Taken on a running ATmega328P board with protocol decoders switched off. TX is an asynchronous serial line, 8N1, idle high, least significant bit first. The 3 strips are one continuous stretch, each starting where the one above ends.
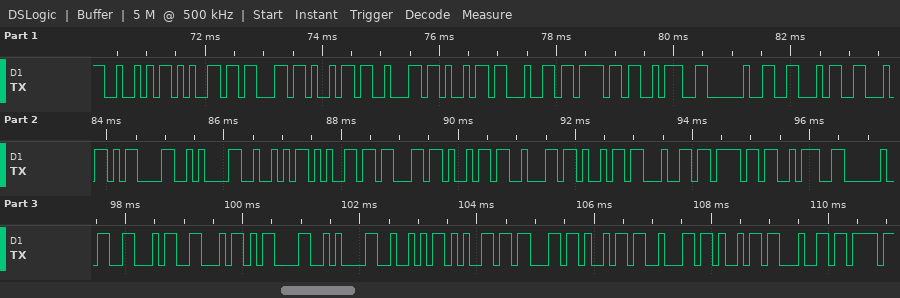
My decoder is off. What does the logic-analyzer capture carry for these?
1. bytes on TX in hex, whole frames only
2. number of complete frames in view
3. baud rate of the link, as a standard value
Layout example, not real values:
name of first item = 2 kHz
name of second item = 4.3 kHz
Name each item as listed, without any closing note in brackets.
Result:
bytes on TX in hex, whole frames only = 0x52 0x65 0x63 0x69 0x62 0x69 0x64 0x6F 0x3A 0x20 0x46 0x46 0x0D 0x0A 0x52 0x65 0x63 0x69 0x62 0x69 0x64 0x6F 0x3A 0x20 0x46 0x46 0x0D 0x0A 0x52 0x65 0x63 0x69 0x62 0x69 0x64
number of complete frames in view = 35
baud rate of the link, as a standard value = 9600 baud
